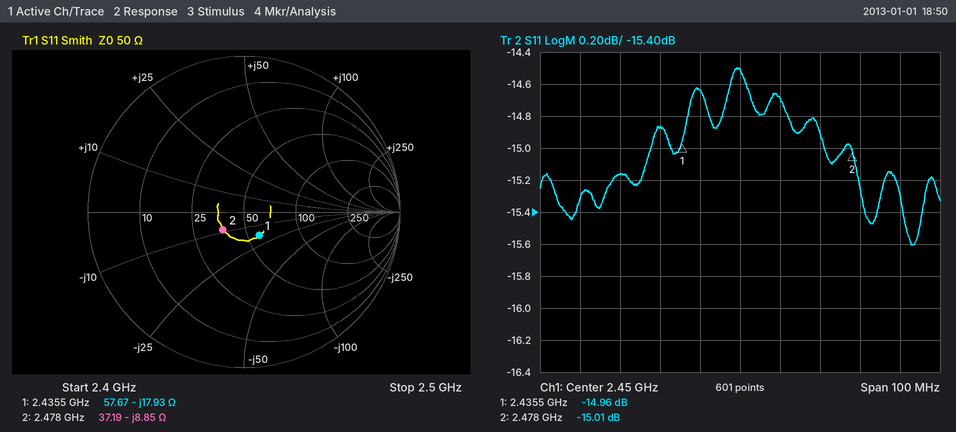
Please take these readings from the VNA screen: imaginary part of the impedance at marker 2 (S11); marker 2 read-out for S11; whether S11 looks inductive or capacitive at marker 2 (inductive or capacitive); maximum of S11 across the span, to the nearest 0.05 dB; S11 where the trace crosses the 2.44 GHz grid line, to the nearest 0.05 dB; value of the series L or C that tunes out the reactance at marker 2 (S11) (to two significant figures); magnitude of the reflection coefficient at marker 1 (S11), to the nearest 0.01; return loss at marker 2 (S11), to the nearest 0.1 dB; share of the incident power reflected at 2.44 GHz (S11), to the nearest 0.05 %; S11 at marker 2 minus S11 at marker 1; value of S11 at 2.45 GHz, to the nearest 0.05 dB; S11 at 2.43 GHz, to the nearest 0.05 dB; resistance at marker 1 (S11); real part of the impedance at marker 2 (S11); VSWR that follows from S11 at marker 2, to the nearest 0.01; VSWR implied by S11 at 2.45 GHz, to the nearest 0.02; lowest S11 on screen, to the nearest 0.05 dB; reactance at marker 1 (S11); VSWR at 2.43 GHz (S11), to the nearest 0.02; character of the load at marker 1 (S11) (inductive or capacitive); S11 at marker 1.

-8.85 Ω
-15.01 dB
capacitive
-14.50 dB
-14.65 dB
570 pH
0.18
15.0 dB
3.45 %
-0.05 dB
-14.50 dB
-14.85 dB
57.67 Ω
37.19 Ω
1.43
1.46
-15.60 dB
-17.93 Ω
1.44
capacitive
-14.96 dB
